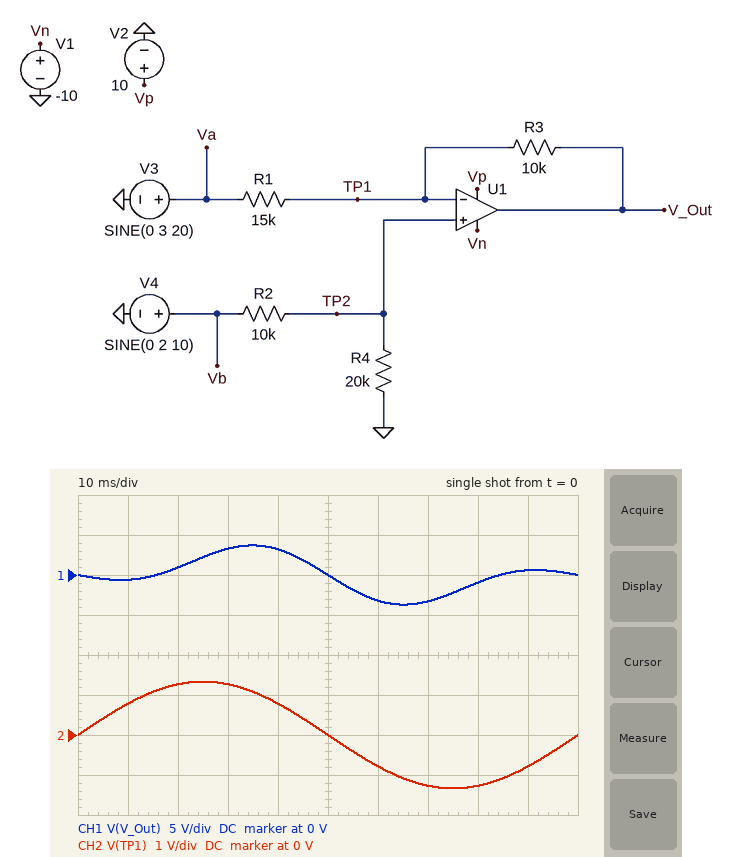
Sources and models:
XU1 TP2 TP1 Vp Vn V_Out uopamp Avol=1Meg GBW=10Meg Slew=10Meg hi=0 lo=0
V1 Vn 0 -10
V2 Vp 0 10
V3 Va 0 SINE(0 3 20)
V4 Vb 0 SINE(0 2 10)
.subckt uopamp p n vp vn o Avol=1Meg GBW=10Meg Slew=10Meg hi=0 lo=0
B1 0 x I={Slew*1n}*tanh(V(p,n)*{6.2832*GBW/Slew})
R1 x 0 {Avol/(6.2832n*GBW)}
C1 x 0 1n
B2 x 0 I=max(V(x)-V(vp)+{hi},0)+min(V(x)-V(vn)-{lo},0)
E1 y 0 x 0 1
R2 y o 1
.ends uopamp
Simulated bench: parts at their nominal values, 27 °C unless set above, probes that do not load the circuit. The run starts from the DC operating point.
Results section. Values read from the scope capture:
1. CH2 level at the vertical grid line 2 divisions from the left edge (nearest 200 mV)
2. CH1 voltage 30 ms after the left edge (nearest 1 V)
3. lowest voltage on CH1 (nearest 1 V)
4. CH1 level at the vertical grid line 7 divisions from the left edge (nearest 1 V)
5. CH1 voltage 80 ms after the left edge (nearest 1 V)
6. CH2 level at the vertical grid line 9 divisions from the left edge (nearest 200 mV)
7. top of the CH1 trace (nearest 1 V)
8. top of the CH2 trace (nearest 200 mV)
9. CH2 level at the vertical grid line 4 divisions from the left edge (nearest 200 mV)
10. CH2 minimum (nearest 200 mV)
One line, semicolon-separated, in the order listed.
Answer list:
1.2 V; 3 V; -4 V; -3 V; -1 V; -800 mV; 4 V; 1.4 V; 800 mV; -1.4 V
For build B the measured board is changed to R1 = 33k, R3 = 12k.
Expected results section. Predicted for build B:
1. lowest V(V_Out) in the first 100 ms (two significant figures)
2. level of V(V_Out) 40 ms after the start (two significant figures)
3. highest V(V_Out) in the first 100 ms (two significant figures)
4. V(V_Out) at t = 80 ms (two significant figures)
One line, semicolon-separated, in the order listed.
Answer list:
-2.5 V; 2.1 V; 2.5 V; -1.1 V
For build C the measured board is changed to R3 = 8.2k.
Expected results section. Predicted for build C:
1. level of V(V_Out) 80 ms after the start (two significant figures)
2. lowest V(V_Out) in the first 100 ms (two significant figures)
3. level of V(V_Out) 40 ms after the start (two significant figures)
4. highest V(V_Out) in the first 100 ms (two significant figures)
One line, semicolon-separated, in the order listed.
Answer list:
-1.0 V; -3.2 V; 2.8 V; 3.2 V
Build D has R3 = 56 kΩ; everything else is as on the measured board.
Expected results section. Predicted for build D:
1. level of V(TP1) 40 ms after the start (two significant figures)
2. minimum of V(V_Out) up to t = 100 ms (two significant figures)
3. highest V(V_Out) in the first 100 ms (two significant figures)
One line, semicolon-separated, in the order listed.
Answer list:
-140 mV; -10 V; 10 V
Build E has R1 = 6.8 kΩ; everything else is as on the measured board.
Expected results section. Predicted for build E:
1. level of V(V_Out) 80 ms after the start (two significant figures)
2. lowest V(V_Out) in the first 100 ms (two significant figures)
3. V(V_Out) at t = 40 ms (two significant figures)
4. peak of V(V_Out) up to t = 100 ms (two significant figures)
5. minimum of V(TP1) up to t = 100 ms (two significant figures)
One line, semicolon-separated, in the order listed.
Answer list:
-540 mV; -6.9 V; 6.1 V; 6.9 V; -1.3 V
